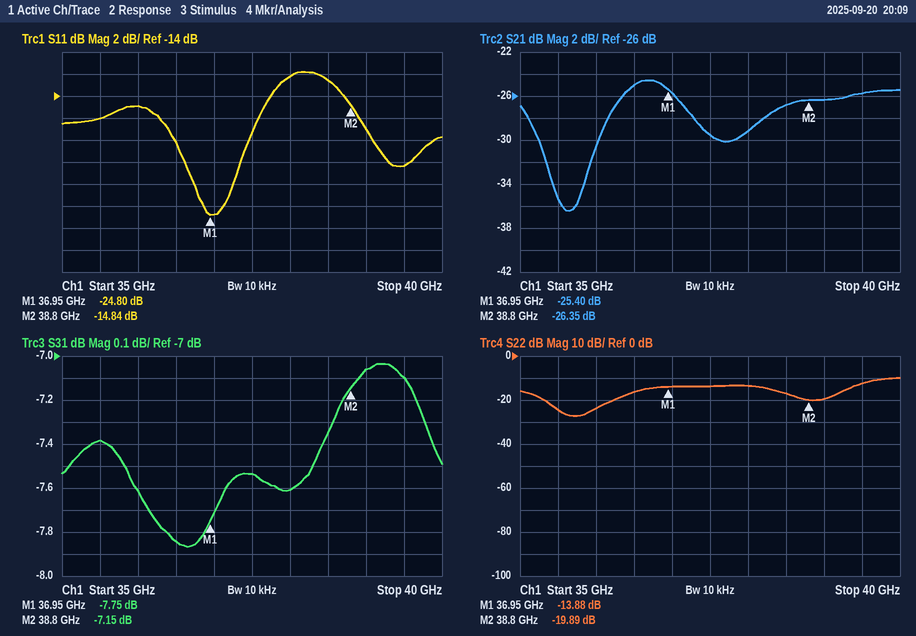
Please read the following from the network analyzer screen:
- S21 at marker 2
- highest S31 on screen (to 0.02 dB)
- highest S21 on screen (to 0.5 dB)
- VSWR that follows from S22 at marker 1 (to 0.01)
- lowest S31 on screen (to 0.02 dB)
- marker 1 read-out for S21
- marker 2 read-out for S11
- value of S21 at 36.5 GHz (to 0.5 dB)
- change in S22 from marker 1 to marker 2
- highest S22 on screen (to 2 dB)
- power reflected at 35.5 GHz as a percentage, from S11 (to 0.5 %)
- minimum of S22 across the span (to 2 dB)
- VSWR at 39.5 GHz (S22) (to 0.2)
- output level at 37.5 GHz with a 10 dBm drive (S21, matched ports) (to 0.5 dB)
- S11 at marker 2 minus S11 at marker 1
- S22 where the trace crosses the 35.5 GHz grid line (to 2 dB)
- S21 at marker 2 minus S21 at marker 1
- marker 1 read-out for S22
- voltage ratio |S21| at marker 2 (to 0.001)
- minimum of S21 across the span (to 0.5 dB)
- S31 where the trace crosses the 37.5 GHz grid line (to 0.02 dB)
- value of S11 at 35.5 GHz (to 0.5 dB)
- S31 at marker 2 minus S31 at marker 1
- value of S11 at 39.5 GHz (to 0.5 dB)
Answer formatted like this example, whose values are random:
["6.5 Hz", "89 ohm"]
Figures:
["-26.35 dB", "-7.04 dB", "-24.5 dB", "1.51", "-7.86 dB", "-25.40 dB", "-14.84 dB", "-25.0 dB", "-6.01 dB", "-10 dB", "2.5 %", "-28 dB", "1.6", "-19.5 dBm", "9.96 dB", "-24 dB", "-0.95 dB", "-13.88 dB", "0.048", "-36.5 dB", "-7.54 dB", "-16.0 dB", "0.60 dB", "-20.5 dB"]
